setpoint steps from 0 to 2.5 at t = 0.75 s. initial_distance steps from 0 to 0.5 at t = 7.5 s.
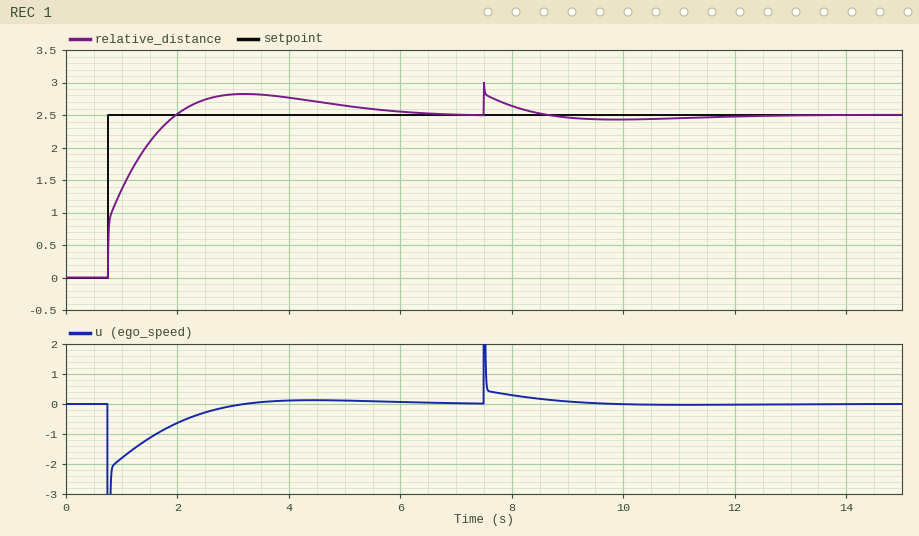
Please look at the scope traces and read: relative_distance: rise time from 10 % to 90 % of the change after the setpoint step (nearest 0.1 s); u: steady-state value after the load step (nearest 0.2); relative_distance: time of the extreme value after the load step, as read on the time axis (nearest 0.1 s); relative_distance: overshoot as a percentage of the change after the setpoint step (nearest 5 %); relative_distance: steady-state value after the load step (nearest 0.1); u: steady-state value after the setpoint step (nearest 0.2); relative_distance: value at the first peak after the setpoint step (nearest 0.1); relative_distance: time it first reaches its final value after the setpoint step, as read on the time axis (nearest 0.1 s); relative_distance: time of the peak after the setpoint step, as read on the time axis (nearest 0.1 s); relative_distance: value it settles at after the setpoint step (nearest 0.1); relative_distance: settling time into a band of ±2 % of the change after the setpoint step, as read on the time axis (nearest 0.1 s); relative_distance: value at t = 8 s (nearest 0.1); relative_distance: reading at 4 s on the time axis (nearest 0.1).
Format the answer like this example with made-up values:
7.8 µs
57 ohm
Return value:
0.9 s
0.0
7.5 s
15 %
2.5
0.0
2.8
2.0 s
3.2 s
2.5
6.0 s
2.6
2.8
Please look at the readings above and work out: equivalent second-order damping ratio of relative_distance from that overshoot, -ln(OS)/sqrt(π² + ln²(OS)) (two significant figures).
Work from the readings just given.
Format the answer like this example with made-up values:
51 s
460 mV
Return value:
0.52
